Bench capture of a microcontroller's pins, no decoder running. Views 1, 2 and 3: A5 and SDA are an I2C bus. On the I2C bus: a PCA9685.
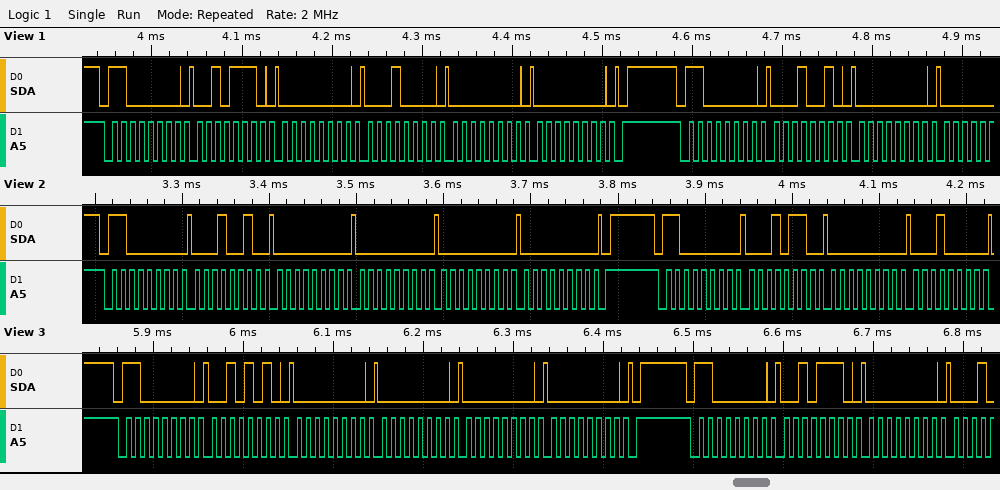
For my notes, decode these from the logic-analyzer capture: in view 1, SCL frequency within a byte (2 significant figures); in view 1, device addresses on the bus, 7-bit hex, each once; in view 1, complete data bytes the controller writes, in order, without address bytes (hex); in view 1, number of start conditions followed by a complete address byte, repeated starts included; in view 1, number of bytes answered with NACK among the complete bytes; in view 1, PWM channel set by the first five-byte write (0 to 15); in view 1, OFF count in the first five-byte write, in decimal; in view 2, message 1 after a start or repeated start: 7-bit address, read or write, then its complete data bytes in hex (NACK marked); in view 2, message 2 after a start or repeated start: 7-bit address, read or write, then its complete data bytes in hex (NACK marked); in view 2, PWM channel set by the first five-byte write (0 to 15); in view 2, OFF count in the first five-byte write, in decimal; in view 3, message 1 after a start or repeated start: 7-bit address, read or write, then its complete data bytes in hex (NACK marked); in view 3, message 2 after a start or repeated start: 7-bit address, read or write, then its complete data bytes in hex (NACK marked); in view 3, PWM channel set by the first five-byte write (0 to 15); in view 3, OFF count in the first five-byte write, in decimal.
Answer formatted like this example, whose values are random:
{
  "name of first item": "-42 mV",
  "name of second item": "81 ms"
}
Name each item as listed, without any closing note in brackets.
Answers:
{
  "in view 1, SCL frequency within a byte": "100 kHz",
  "in view 1, device addresses on the bus, 7-bit hex, each once": "0x60",
  "in view 1, complete data bytes the controller writes, in order, without address bytes": "2E 00 10 00 00 12 00",
  "in view 1, number of start conditions followed by a complete address byte, repeated starts included": "2",
  "in view 1, number of bytes answered with NACK among the complete bytes": "0",
  "in view 1, PWM channel set by the first five-byte write": "10",
  "in view 1, OFF count in the first five-byte write, in decimal": "0",
  "in view 2, message 1 after a start or repeated start: 7-bit address, read or write, then its complete data bytes in hex": "0x60 write: 12 00 00 00 00",
  "in view 2, message 2 after a start or repeated start: 7-bit address, read or write, then its complete data bytes in hex": "0x60 write: 16 00 10",
  "in view 2, PWM channel set by the first five-byte write": "3",
  "in view 2, OFF count in the first five-byte write, in decimal": "0",
  "in view 3, message 1 after a start or repeated start: 7-bit address, read or write, then its complete data bytes in hex": "0x60 write: 2A 00 00 00 00",
  "in view 3, message 2 after a start or repeated start: 7-bit address, read or write, then its complete data bytes in hex": "0x60 write: 2E 00",
  "in view 3, PWM channel set by the first five-byte write": "9",
  "in view 3, OFF count in the first five-byte write, in decimal": "0"
}
